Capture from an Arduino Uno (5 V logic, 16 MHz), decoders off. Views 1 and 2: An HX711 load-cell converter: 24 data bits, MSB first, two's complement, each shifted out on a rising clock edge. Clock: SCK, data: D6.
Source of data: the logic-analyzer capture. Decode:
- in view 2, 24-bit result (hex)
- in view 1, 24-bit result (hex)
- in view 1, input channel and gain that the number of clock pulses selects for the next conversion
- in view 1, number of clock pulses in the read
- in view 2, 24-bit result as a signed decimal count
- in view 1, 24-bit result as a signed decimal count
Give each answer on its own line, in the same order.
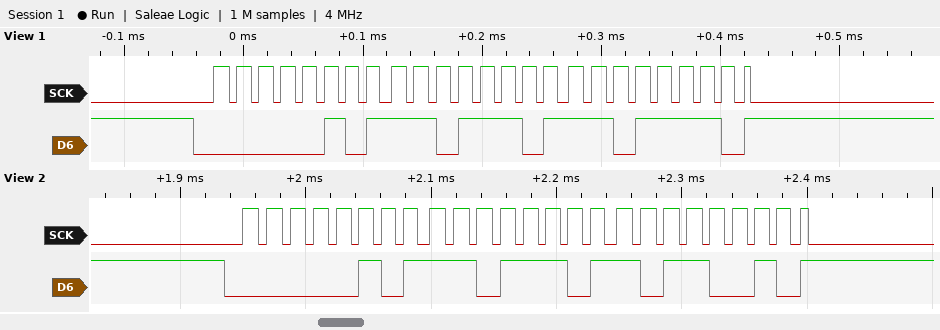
0x05DDB2
0x05DDDE
channel A, gain 128
25
384434
384478
